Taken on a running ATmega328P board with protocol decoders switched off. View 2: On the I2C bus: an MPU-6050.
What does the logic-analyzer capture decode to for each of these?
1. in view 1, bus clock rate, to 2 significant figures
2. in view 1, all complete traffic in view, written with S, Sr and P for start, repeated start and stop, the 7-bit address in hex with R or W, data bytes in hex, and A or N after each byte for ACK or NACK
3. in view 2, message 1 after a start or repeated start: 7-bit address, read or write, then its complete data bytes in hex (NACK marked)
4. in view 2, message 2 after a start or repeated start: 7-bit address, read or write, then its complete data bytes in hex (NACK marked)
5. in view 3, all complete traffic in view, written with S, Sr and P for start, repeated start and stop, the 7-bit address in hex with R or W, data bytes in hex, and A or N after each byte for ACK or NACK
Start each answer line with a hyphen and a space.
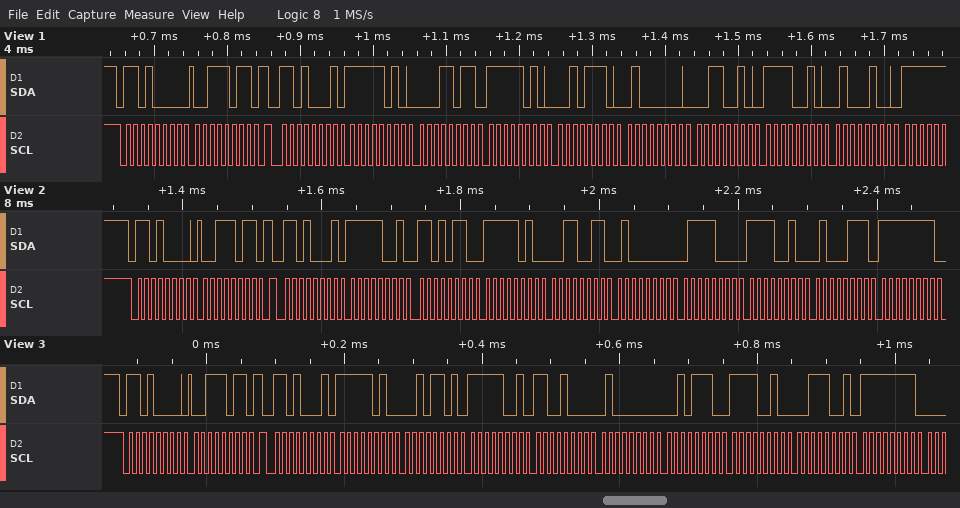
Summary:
- 100 kHz
- S 68W A 3B A Sr 68R A FA A 1B A FA A 2E A 40 A 32 A F2 A 44 A
- 0x68 write: 3B
- 0x68 read: F9 D6 FA 33 40 78 F2 47 FF
- S 68W A 3B A Sr 68R A FA A 2D A F9 A C8 A 40 A 2E A F2 A 39 A FF A
